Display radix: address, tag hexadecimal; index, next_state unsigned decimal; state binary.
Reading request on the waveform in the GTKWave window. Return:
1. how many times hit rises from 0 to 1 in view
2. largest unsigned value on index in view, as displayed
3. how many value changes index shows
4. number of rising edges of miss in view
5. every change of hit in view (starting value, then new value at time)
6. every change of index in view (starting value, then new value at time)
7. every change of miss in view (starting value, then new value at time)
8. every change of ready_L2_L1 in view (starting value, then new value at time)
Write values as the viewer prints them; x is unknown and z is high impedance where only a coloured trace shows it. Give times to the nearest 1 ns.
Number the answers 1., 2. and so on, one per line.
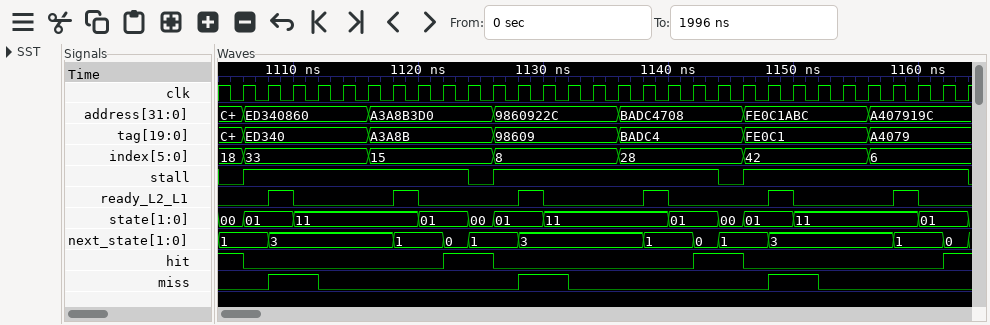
1. 3
2. 42
3. 6
4. 3
5. 1, 0 at 1106 ns, 1 at 1122 ns, 0 at 1126 ns, 1 at 1142 ns, 0 at 1146 ns, 1 at 1162 ns
6. 18, 33 at 1106 ns, 15 at 1116 ns, 8 at 1126 ns, 28 at 1136 ns, 42 at 1146 ns, 6 at 1156 ns
7. 0, 1 at 1108 ns, 0 at 1112 ns, 1 at 1128 ns, 0 at 1132 ns, 1 at 1148 ns, 0 at 1152 ns
8. 0, 1 at 1108 ns, 0 at 1110 ns, 1 at 1118 ns, 0 at 1120 ns, 1 at 1128 ns, 0 at 1130 ns, 1 at 1138 ns, 0 at 1140 ns, 1 at 1148 ns, 0 at 1150 ns, 1 at 1158 ns, 0 at 1160 ns
